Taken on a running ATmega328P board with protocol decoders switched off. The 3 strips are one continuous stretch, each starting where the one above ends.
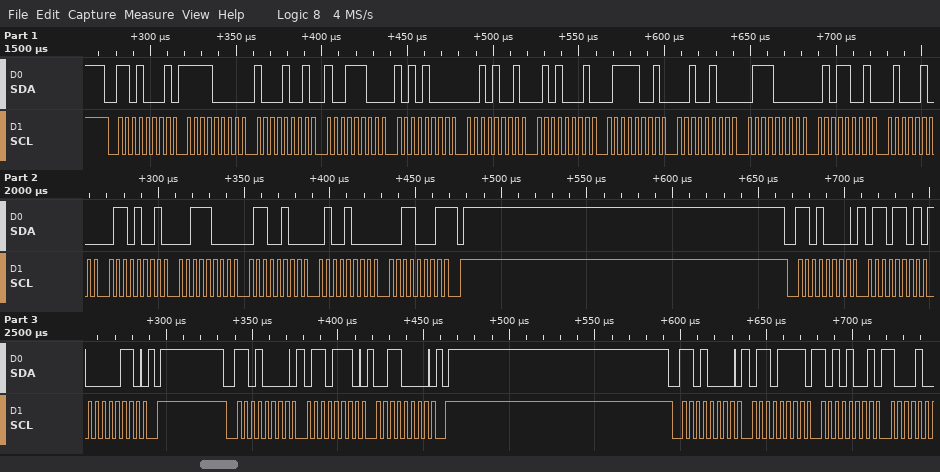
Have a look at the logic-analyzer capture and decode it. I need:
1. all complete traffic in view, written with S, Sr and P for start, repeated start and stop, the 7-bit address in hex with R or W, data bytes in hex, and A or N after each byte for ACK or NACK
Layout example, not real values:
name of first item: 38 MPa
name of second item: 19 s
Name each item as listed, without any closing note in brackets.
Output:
all complete traffic in view, written with S, Sr and P for start, repeated start and stop, the 7-bit address in hex with R or W, data bytes in hex, and A or N after each byte for ACK or NACK: S 68R A F0 A 89 A 9C A A8 A 29 A 51 A 79 A 24 A 70 A 59 A 44 A 69 A 38 A 64 A 48 A 31 N P S 68W A 6D A 06 A P S 68W A 6E A 30 A P S 68W A 6F A A9 A
